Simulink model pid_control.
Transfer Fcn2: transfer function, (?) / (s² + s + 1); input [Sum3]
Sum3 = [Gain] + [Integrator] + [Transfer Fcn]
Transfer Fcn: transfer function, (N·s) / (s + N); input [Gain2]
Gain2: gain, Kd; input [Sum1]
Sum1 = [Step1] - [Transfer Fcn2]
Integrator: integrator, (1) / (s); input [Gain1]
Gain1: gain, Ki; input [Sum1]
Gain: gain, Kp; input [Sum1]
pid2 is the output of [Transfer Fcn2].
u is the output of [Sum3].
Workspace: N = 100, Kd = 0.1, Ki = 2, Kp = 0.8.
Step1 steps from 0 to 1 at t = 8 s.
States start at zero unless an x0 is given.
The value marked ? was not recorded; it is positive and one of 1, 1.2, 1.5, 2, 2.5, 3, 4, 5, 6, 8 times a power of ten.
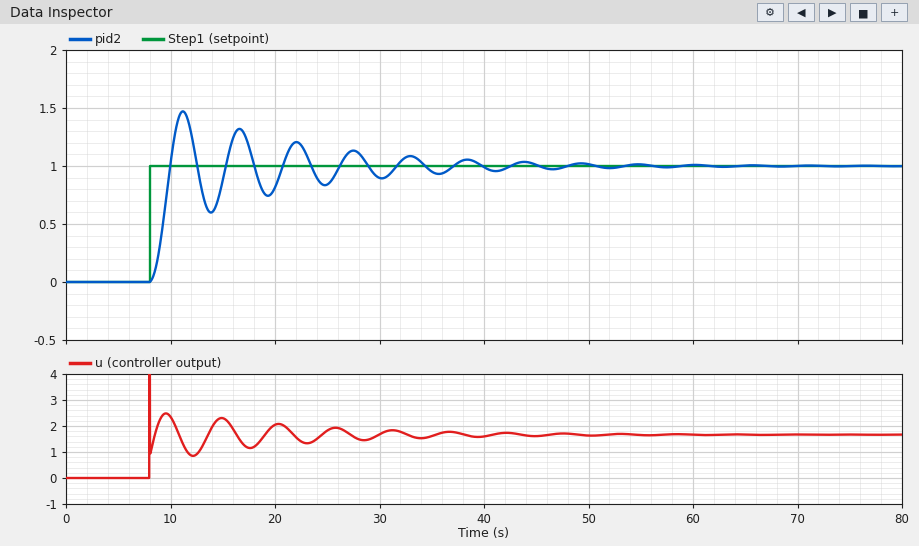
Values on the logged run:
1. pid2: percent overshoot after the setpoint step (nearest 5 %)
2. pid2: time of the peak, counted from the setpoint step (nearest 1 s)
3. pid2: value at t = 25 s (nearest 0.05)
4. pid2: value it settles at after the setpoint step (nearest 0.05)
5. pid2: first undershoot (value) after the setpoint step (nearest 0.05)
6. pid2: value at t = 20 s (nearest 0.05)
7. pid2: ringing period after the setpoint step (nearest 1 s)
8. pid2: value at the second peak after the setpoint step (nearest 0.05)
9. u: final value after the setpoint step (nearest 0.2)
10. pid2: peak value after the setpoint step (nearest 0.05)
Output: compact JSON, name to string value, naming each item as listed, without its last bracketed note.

{"pid2: percent overshoot after the setpoint step": "45 %", "pid2: time of the peak, counted from the setpoint step": "3 s", "pid2: value at t = 25 s": "0.85", "pid2: value it settles at after the setpoint step": "1.00", "pid2: first undershoot (value) after the setpoint step": "0.60", "pid2: value at t = 20 s": "0.80", "pid2: ringing period after the setpoint step": "5 s", "pid2: value at the second peak after the setpoint step": "1.30", "u: final value after the setpoint step": "1.6", "pid2: peak value after the setpoint step": "1.45"}
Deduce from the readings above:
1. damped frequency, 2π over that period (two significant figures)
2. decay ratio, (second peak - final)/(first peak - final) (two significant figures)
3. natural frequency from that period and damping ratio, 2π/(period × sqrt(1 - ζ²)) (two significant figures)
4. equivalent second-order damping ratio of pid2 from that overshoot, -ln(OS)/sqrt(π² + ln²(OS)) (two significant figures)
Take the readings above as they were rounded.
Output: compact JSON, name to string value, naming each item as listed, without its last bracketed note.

{"damped frequency, 2π over that period": "1.3 rad/s", "decay ratio, (second peak - final)/(first peak - final)": "0.67", "natural frequency from that period and damping ratio, 2π/(period × sqrt(1 - ζ²))": "1.3 rad/s", "equivalent second-order damping ratio of pid2 from that overshoot, -ln(OS)/sqrt(π² + ln²(OS))": "0.25"}
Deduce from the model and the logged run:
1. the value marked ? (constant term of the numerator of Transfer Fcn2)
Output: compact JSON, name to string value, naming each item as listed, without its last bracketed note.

{"the value marked ?": "0.6"}
